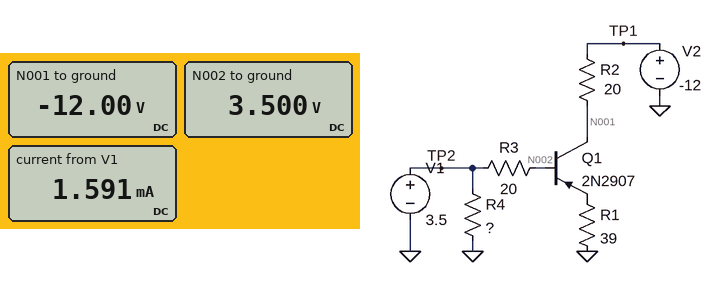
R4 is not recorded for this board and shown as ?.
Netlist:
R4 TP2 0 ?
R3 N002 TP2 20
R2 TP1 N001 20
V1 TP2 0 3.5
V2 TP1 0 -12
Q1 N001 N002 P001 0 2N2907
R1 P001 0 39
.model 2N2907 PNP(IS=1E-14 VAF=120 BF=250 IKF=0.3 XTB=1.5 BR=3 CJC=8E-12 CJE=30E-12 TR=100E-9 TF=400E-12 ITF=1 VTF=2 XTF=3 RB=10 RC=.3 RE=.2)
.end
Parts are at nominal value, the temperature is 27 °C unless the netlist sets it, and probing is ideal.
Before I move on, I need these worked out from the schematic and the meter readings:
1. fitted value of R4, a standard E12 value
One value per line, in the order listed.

2.2 kΩ
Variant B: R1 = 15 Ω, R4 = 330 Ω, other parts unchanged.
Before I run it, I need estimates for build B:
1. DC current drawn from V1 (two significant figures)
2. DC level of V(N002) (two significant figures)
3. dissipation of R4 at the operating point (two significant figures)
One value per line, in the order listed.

11 mA
3.5 V
37 mW
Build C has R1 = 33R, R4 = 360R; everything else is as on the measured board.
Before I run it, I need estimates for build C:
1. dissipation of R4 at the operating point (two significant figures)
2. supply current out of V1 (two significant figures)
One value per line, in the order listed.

34 mW
9.7 mA
